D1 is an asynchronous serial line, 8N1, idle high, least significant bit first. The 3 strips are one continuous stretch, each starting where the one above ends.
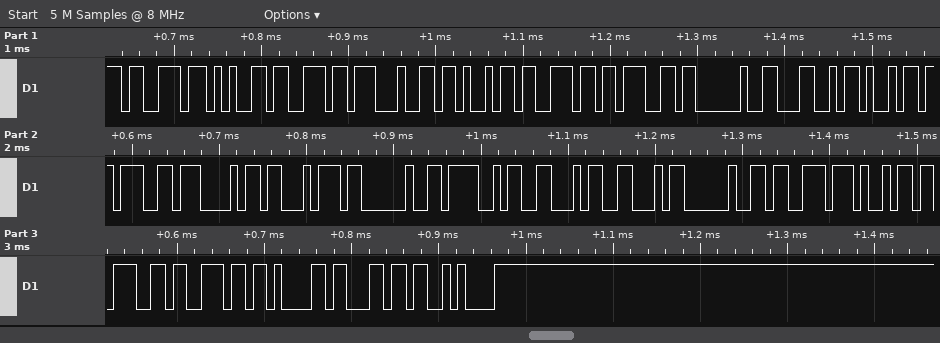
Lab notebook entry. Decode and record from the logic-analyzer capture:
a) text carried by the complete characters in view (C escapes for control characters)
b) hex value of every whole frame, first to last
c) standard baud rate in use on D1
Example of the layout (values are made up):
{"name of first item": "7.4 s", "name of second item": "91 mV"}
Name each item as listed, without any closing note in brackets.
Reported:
{"text carried by the complete characters in view": "\"sending Light OFF signal\\n\"", "hex value of every whole frame, first to last": "73 65 6E 64 69 6E 67 20 4C 69 67 68 74 20 4F 46 46 20 73 69 67 6E 61 6C 0A", "standard baud rate in use on D1": "115200 baud"}
